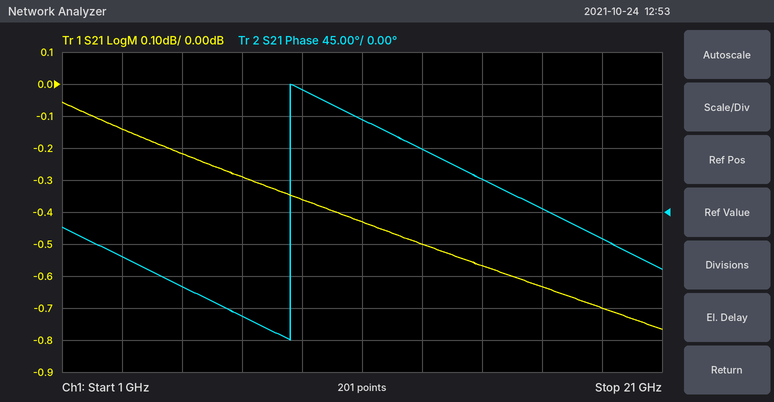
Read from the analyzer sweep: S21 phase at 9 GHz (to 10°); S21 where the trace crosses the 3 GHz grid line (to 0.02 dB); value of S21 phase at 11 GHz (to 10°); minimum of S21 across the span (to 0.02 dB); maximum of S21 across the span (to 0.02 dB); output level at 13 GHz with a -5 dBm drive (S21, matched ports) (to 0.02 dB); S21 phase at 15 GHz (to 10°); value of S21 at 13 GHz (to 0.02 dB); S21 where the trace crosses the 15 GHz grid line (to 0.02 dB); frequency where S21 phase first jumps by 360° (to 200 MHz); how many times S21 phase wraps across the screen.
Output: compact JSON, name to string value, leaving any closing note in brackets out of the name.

{"S21 phase at 9 GHz": "170°", "S21 where the trace crosses the 3 GHz grid line": "-0.14 dB", "value of S21 phase at 11 GHz": "130°", "minimum of S21 across the span": "-0.76 dB", "maximum of S21 across the span": "-0.06 dB", "output level at 13 GHz with a -5 dBm drive (S21, matched ports)": "-5.50 dBm", "S21 phase at 15 GHz": "50°", "value of S21 at 13 GHz": "-0.50 dB", "S21 where the trace crosses the 15 GHz grid line": "-0.56 dB", "frequency where S21 phase first jumps by 360°": "8.6 GHz", "how many times S21 phase wraps across the screen": "1"}
